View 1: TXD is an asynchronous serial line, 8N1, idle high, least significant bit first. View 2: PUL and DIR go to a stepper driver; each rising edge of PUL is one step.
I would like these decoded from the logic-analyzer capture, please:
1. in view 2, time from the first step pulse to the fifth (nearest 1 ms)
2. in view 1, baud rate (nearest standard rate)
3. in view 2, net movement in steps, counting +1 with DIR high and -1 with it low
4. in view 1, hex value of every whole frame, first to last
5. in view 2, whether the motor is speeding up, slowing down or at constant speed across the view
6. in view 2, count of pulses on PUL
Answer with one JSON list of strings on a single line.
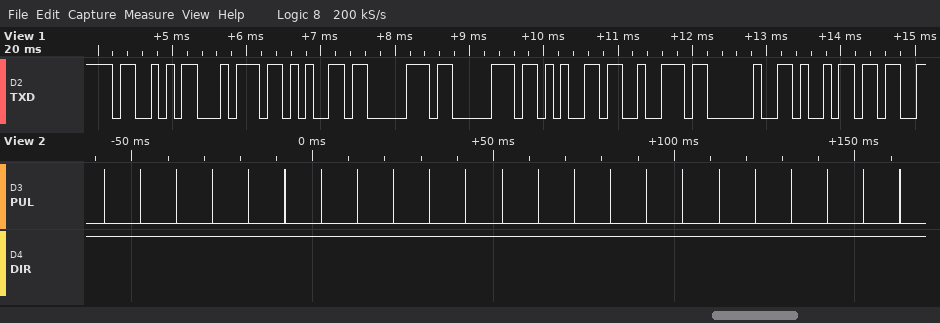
["40 ms", "9600 baud", "+23", "0x53 0x74 0x65 0x70 0x70 0x65 0x72 0x20 0x69", "constant speed", "23"]
